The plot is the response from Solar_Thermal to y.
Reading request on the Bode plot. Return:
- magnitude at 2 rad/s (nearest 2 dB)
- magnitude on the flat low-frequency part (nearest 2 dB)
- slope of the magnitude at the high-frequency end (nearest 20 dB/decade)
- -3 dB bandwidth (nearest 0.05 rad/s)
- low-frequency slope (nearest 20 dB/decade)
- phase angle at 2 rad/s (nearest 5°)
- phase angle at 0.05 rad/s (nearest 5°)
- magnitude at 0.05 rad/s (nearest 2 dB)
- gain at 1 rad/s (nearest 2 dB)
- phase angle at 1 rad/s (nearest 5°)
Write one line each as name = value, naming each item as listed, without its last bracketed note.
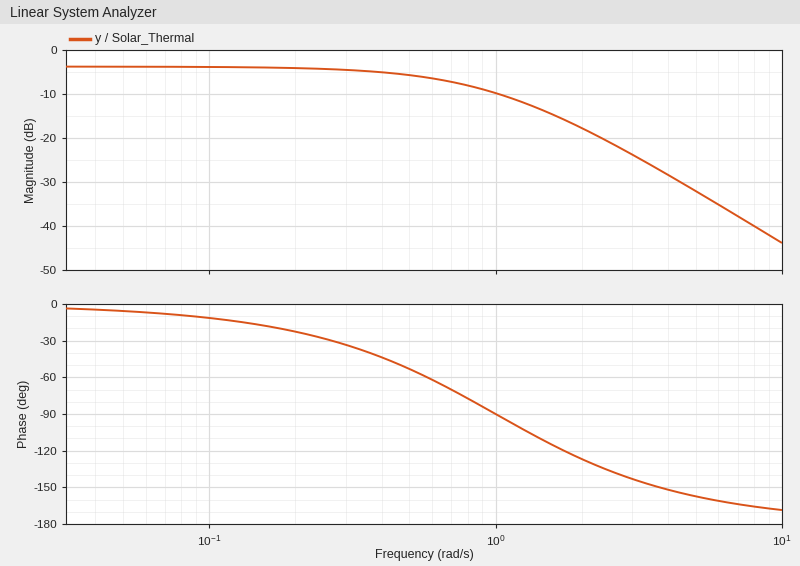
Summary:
magnitude at 2 rad/s = -18 dB
magnitude on the flat low-frequency part = -4 dB
slope of the magnitude at the high-frequency end = -40 dB/decade
-3 dB bandwidth = 0.65 rad/s
low-frequency slope = 0 dB/decade
phase angle at 2 rad/s = -125°
phase angle at 0.05 rad/s = -5°
magnitude at 0.05 rad/s = -4 dB
gain at 1 rad/s = -10 dB
phase angle at 1 rad/s = -90°
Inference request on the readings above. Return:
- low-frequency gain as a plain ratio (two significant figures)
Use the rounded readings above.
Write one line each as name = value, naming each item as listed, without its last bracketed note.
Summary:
low-frequency gain as a plain ratio = 0.63
